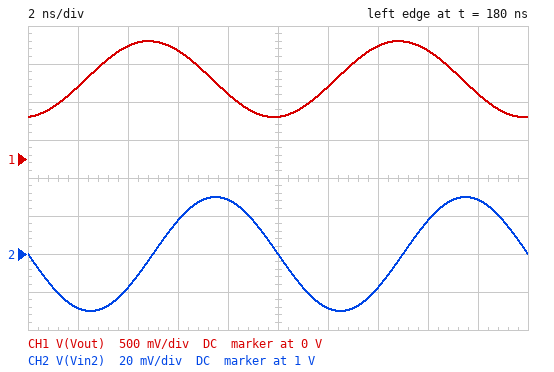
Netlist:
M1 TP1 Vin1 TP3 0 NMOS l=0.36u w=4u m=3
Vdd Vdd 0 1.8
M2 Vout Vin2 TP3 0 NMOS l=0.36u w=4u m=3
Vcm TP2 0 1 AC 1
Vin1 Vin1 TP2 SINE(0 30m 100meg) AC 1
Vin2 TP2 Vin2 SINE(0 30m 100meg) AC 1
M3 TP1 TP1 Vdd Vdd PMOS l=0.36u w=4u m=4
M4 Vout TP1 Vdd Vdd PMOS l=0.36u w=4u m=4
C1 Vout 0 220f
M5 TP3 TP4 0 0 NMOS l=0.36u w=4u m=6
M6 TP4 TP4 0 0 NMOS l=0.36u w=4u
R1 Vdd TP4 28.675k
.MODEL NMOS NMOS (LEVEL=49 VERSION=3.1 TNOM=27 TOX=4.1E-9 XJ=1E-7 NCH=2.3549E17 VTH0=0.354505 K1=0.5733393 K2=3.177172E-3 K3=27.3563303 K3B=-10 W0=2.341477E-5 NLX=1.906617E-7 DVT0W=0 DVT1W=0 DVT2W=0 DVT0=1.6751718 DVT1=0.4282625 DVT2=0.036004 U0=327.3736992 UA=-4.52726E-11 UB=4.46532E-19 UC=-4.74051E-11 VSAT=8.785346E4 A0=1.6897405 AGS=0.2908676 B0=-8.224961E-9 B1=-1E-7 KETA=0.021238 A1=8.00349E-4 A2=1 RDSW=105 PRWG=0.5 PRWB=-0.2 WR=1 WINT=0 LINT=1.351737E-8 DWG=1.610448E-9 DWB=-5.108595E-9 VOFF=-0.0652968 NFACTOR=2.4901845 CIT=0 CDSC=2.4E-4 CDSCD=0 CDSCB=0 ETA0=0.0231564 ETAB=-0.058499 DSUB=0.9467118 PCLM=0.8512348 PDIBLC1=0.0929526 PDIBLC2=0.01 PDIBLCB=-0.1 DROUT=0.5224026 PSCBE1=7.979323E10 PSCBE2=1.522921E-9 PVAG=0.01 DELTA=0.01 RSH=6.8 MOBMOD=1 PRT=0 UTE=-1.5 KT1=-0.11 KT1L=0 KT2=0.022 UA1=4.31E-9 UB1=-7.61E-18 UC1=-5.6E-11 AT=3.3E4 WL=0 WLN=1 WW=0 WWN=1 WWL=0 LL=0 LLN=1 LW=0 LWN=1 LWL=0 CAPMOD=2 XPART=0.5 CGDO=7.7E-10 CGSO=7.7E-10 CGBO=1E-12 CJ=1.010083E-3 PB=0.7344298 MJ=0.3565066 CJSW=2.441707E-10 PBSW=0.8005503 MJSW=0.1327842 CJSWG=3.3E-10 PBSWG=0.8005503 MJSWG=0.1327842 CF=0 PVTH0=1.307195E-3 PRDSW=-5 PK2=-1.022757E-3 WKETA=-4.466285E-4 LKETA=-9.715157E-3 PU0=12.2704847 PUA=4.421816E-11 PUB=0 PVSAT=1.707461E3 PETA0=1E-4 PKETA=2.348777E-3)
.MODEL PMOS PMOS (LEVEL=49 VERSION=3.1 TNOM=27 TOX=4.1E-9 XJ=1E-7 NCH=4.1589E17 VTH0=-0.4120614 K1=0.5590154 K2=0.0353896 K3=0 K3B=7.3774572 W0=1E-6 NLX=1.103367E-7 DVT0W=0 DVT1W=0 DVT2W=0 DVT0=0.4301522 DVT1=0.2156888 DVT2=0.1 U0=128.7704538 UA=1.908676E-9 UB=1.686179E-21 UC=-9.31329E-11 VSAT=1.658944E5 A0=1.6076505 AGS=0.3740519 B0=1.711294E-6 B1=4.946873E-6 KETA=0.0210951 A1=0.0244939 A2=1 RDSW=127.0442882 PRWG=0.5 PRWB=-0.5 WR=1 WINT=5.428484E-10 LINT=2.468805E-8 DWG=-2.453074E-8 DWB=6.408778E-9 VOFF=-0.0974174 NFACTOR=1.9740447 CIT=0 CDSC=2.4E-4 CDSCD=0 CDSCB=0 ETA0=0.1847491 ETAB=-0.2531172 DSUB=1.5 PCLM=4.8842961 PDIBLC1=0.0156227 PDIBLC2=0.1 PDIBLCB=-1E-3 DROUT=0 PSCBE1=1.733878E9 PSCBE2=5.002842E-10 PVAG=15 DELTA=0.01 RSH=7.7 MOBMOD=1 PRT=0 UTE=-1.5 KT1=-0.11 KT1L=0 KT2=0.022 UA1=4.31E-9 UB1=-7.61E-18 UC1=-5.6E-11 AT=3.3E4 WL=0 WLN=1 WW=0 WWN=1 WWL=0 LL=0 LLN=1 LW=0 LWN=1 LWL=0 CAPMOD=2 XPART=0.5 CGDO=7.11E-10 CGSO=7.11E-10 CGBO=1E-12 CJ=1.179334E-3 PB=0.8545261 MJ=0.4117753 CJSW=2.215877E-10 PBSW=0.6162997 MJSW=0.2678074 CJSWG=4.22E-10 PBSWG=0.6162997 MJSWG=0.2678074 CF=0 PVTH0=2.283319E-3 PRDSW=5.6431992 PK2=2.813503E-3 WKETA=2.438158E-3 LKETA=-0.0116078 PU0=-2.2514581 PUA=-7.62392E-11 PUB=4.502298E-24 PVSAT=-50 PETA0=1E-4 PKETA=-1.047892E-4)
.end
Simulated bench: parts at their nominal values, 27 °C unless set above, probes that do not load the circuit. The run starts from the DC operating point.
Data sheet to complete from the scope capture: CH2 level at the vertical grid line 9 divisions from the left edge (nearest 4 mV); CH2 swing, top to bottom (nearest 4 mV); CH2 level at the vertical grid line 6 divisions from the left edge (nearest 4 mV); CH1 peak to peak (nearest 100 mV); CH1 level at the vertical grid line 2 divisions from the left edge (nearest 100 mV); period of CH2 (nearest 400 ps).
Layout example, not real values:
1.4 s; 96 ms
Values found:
1.028 V; 60 mV; 972 mV; 1.0 V; 1.5 V; 10.0 ns
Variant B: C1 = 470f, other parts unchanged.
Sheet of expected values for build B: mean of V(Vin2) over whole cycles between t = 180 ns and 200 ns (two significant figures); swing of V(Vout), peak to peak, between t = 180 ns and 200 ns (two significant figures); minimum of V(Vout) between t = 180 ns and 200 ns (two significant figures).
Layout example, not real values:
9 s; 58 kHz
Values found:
1.0 V; 510 mV; 800 mV
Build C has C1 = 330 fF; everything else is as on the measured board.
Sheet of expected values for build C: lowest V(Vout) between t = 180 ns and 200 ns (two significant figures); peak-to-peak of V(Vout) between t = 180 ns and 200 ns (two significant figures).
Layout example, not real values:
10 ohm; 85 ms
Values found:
700 mV; 710 mV
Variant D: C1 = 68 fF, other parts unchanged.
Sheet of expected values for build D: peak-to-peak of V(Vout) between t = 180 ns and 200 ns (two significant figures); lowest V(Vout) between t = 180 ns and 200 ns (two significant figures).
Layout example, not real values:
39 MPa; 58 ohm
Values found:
1.4 V; 330 mV
